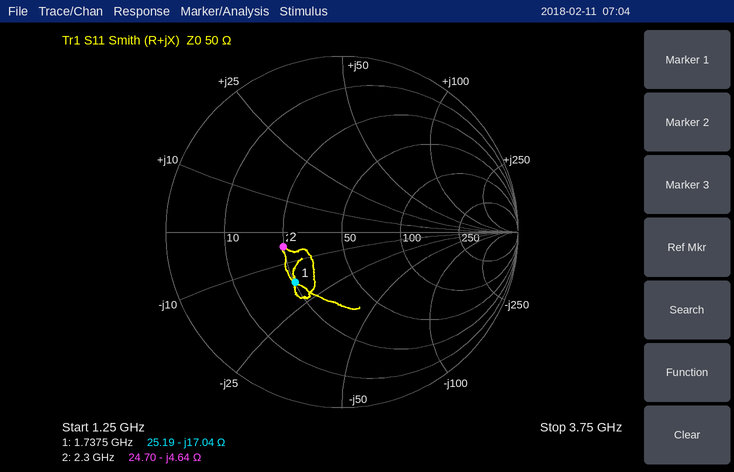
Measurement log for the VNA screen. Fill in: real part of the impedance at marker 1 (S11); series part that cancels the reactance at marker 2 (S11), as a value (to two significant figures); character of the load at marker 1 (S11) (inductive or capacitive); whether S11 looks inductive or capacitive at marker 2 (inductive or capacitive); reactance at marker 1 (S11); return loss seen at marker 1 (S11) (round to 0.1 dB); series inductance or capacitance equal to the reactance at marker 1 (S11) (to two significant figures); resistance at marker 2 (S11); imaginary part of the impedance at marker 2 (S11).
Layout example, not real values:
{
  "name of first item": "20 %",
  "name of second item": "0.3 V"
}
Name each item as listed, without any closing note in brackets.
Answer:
{
  "real part of the impedance at marker 1": "25.19 Ω",
  "series part that cancels the reactance at marker 2 (S11), as a value": "320 pH",
  "character of the load at marker 1 (S11)": "capacitive",
  "whether S11 looks inductive or capacitive at marker 2": "capacitive",
  "reactance at marker 1": "-17.04 Ω",
  "return loss seen at marker 1 (S11)": "8.2 dB",
  "series inductance or capacitance equal to the reactance at marker 1 (S11)": "5.4 pF",
  "resistance at marker 2": "24.70 Ω",
  "imaginary part of the impedance at marker 2": "-4.64 Ω"
}
